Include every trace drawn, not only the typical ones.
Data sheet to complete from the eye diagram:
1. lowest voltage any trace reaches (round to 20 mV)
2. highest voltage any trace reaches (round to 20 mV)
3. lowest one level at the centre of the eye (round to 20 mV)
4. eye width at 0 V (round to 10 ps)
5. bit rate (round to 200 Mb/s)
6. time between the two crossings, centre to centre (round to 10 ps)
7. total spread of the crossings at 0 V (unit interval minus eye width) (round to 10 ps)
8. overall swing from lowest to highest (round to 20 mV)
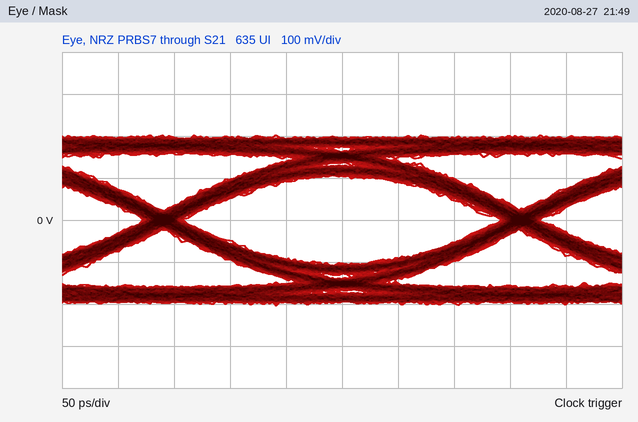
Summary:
-200 mV
200 mV
100 mV
280 ps
3.2 Gb/s
320 ps
40 ps
400 mV
